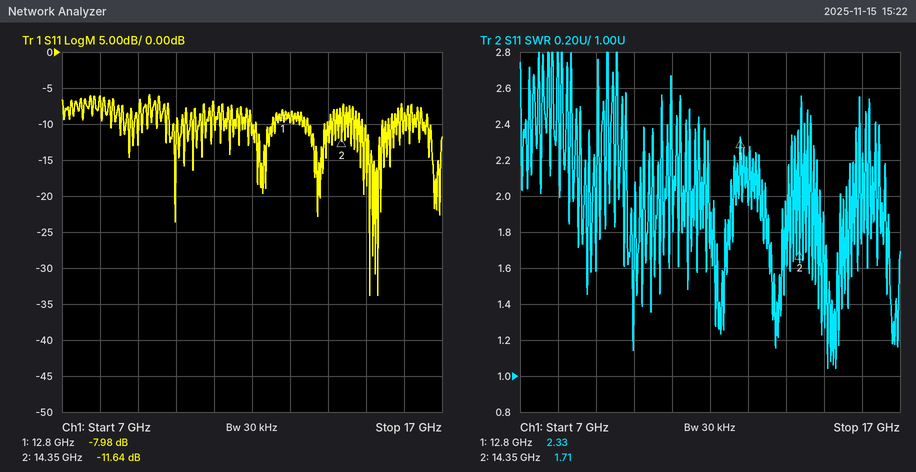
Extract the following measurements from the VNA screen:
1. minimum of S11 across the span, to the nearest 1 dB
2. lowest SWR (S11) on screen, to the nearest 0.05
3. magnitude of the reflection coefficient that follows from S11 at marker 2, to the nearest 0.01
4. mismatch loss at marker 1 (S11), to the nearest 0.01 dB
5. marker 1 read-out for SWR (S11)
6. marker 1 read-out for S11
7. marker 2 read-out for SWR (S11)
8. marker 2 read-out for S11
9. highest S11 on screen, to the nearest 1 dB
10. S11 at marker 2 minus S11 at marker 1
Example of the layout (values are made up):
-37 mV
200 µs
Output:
-34 dB
1.05
0.26
0.75 dB
2.33
-7.98 dB
1.71
-11.64 dB
-6 dB
-3.66 dB
